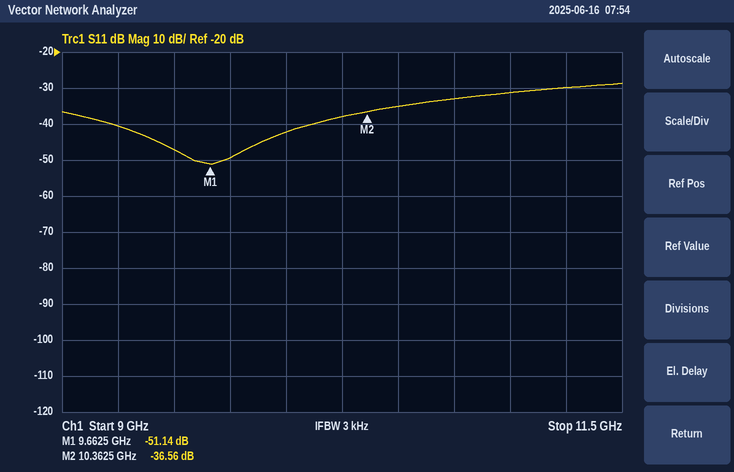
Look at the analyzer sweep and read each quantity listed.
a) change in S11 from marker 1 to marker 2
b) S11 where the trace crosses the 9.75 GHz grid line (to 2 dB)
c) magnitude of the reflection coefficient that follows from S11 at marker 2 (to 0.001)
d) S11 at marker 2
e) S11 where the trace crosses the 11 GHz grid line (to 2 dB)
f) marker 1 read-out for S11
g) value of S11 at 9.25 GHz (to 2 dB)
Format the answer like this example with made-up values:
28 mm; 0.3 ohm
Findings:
14.58 dB; -50 dB; 0.015; -36.56 dB; -32 dB; -51.14 dB; -40 dB
